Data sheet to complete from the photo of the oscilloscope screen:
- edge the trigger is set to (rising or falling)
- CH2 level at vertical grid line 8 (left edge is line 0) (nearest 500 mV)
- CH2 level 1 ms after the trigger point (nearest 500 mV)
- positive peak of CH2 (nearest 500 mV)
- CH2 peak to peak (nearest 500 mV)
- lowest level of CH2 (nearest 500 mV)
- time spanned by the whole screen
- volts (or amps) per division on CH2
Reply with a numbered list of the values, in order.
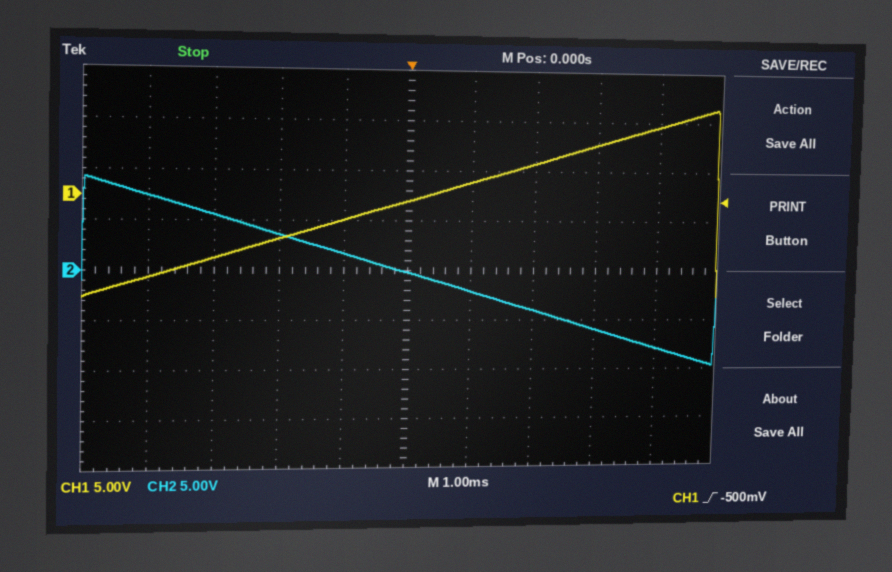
1. rising
2. -6.0 V
3. -2.0 V
4. 9.5 V
5. 19.0 V
6. -9.5 V
7. 10 ms
8. 5 V
